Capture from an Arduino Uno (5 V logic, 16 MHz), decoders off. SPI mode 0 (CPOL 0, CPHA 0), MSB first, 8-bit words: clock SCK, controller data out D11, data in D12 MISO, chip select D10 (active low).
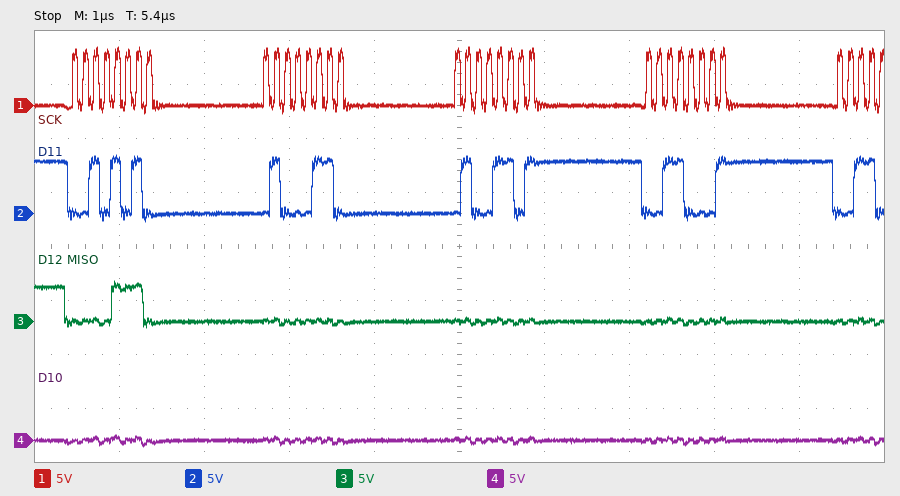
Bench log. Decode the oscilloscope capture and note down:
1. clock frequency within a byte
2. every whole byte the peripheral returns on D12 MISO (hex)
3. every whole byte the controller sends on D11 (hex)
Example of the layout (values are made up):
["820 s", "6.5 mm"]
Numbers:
["8 MHz", "0x0E 0x00 0x00 0x00", "0x2A 0x46 0x4D 0x31"]
